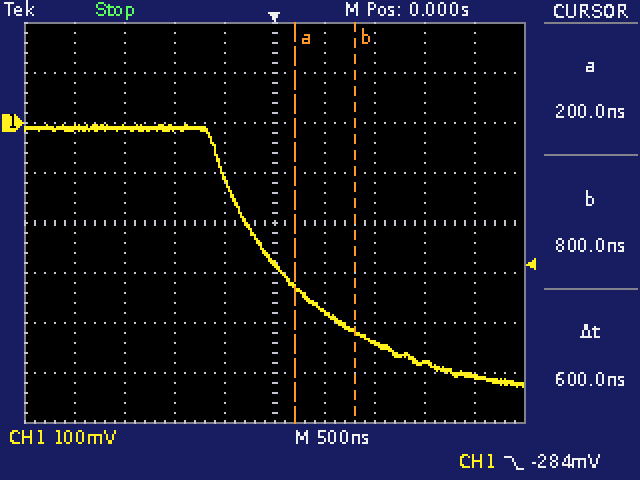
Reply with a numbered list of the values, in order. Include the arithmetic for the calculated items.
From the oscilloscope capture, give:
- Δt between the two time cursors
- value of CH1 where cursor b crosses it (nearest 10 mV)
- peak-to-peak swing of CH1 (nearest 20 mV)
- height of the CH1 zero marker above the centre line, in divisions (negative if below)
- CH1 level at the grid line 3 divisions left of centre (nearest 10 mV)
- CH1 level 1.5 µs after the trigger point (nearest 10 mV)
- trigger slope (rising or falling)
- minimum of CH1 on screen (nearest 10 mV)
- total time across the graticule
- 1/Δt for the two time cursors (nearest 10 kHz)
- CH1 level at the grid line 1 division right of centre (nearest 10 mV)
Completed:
1. 600 ns
2. -420 mV
3. 520 mV
4. +2.0 div
5. -10 mV
6. -480 mV
7. falling
8. -530 mV
9. 5 µs
10. 1 / 600 ns ≈ 1.67 MHz
11. -380 mV
